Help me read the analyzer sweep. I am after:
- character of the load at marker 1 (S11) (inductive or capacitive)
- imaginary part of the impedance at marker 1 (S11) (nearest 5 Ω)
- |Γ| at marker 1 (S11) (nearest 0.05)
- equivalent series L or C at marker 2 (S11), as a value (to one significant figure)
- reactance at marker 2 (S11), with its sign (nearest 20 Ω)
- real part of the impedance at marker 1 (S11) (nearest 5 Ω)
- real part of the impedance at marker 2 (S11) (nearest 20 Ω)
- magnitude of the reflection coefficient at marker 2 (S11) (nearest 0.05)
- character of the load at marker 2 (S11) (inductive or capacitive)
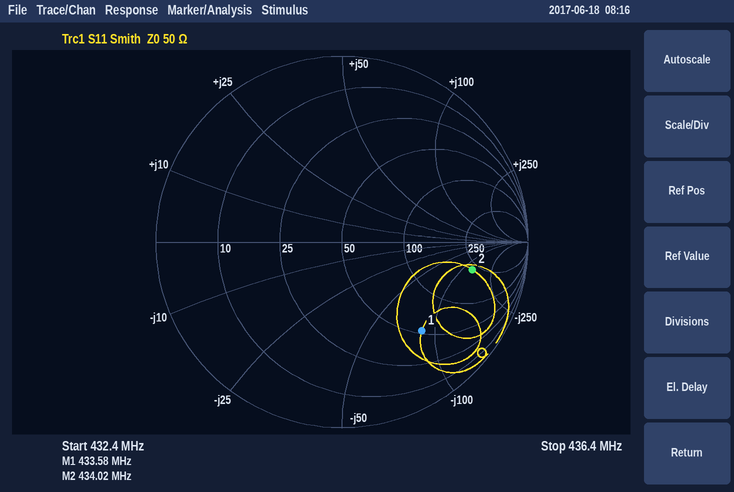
capacitive
-85 Ω
0.65
3 pF
-140 Ω
55 Ω
220 Ω
0.70
capacitive
